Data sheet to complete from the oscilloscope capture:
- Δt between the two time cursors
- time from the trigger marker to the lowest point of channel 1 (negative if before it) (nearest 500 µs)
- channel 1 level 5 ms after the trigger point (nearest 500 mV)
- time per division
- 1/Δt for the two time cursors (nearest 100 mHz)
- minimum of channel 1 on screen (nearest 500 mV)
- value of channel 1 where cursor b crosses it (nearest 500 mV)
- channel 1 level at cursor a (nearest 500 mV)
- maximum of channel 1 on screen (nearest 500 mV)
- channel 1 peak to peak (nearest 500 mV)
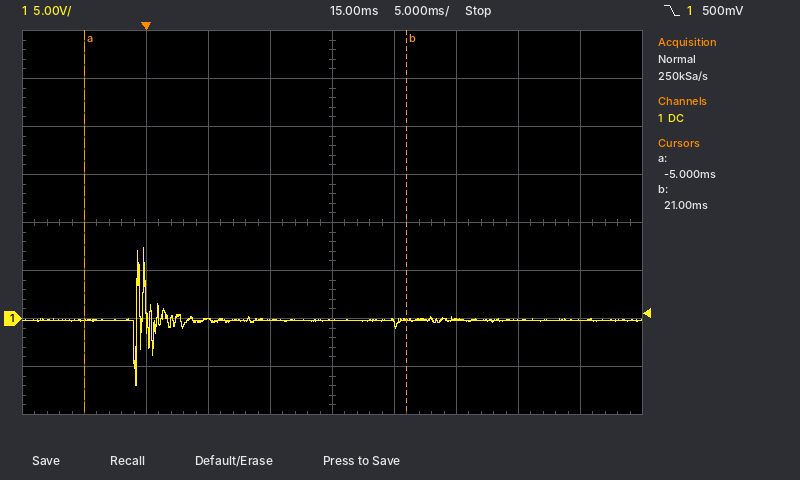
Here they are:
26.0 ms
-1.0 ms
0.0 V
5 ms
38.5 Hz
-7.0 V
0.0 V
0.0 V
7.5 V
14.5 V
